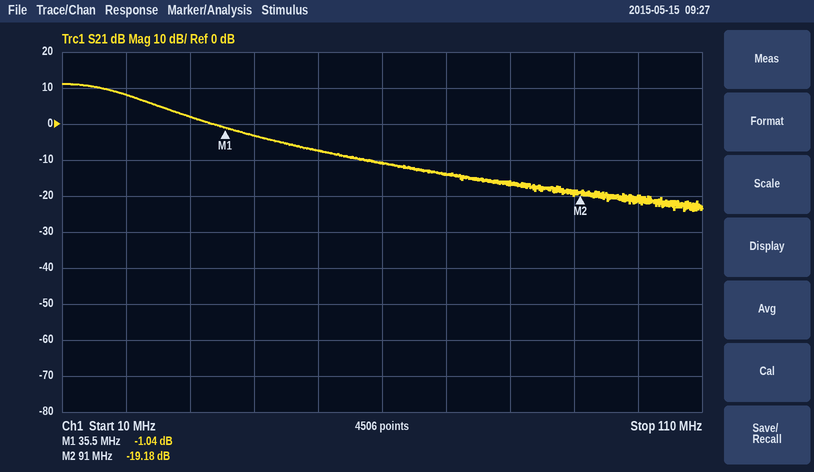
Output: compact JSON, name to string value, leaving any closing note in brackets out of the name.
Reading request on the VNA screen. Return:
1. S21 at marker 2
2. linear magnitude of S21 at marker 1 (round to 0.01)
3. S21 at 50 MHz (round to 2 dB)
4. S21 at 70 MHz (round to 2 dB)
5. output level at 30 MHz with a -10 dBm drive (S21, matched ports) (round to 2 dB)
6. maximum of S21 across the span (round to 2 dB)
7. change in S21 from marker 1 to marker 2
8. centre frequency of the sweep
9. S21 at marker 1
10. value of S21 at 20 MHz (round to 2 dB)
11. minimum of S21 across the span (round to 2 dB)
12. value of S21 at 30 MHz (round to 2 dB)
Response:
{"S21 at marker 2": "-19.18 dB", "linear magnitude of S21 at marker 1": "0.89", "S21 at 50 MHz": "-8 dB", "S21 at 70 MHz": "-14 dB", "output level at 30 MHz with a -10 dBm drive (S21, matched ports)": "-8 dBm", "maximum of S21 across the span": "12 dB", "change in S21 from marker 1 to marker 2": "-18.14 dB", "centre frequency of the sweep": "60 MHz", "S21 at marker 1": "-1.04 dB", "value of S21 at 20 MHz": "8 dB", "minimum of S21 across the span": "-24 dB", "value of S21 at 30 MHz": "2 dB"}
